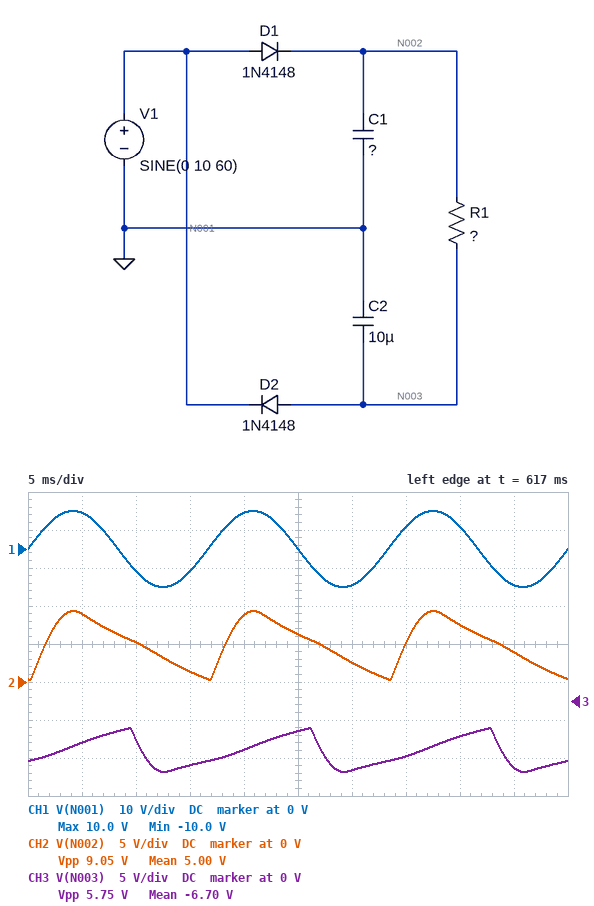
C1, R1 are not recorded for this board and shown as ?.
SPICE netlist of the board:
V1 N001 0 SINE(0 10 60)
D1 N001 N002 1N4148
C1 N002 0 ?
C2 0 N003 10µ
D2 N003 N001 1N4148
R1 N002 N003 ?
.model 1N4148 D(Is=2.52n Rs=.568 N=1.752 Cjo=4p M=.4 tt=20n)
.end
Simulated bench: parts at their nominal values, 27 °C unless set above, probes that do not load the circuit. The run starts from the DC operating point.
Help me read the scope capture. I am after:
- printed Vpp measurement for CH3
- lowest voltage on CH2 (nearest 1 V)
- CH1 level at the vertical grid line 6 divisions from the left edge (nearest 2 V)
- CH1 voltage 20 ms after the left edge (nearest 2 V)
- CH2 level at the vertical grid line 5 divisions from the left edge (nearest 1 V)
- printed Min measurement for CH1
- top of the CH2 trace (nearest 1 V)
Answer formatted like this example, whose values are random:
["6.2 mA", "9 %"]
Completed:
["5.75 V", "0 V", "-10 V", "10 V", "6 V", "-10.0 V", "9 V"]
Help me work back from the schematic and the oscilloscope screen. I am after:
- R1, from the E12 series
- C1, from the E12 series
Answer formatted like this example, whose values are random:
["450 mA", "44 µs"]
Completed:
["2.7 kΩ", "5.6 µF"]
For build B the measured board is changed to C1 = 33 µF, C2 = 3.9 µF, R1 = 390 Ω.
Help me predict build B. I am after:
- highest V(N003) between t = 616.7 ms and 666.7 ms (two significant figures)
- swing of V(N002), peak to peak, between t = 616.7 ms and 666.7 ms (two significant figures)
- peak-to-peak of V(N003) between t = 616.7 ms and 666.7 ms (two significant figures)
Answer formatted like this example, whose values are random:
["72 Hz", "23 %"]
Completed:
["8.5 V", "7.7 V", "18 V"]
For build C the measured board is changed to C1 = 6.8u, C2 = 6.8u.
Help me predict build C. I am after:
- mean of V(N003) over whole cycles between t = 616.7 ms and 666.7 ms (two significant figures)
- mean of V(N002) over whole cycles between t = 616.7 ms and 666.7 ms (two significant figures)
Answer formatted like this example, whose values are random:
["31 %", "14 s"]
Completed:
["-5.7 V", "5.7 V"]
